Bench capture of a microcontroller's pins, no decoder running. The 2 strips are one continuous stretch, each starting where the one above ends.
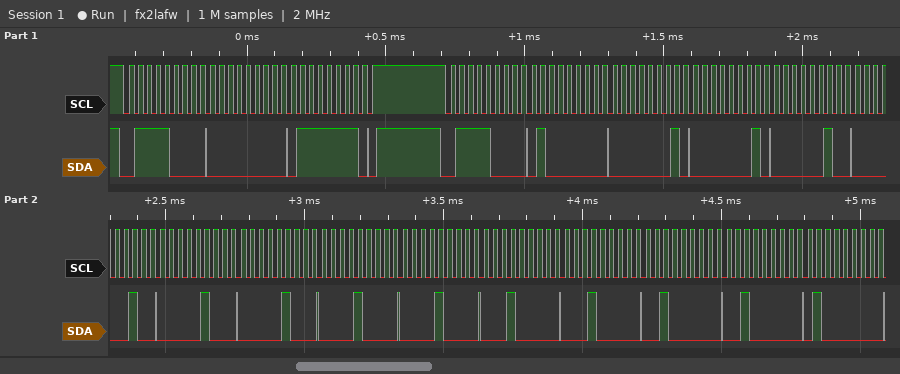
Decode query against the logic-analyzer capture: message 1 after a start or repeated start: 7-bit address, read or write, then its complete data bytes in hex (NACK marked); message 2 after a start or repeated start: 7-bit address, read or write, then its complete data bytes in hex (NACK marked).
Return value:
0x3C write: 00 7F
0x3C write: 40 01 01 02 02 04 04 08 08 10 10 20 20 40
